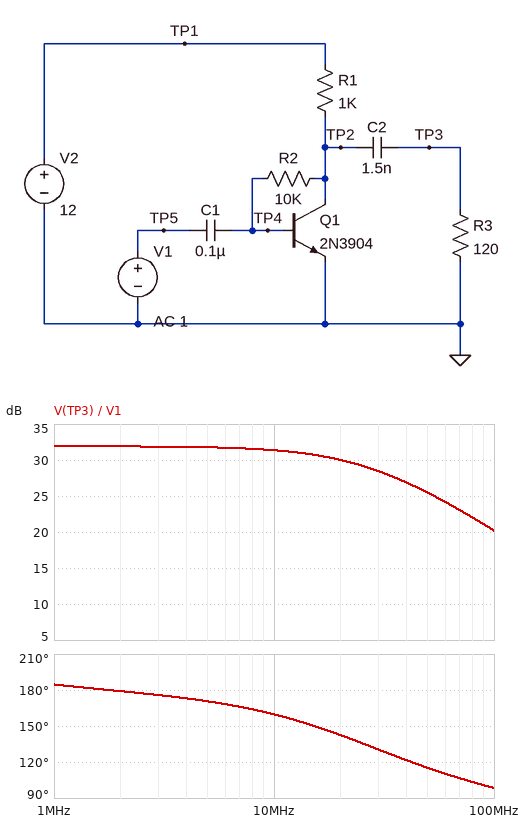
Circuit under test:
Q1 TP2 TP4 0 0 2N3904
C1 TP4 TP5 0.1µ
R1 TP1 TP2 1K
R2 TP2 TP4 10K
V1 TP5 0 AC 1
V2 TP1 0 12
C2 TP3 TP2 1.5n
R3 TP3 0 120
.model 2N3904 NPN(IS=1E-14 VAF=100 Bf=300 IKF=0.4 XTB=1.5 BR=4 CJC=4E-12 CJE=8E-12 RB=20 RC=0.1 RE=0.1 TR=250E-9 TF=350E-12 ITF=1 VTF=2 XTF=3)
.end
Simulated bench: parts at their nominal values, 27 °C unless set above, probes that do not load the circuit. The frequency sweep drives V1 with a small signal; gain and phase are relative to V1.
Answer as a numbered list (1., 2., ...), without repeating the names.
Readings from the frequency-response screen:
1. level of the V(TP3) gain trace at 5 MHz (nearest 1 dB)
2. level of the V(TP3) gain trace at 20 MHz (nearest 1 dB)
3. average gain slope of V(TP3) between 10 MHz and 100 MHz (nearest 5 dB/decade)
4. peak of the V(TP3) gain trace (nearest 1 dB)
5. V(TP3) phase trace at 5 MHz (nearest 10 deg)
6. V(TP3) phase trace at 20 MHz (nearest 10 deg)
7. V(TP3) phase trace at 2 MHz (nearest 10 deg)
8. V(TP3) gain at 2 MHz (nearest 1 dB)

1. 32 dB
2. 30 dB
3. -10 dB/decade
4. 32 dB
5. 170 deg
6. 140 deg
7. 180 deg
8. 32 dB
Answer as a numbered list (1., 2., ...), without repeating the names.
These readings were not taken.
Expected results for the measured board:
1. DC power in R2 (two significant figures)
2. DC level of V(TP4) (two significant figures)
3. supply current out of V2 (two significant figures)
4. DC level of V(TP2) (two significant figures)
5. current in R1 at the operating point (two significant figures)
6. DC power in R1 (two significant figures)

1. 14 µW
2. 720 mV
3. 11 mA
4. 1.1 V
5. 11 mA
6. 120 mW
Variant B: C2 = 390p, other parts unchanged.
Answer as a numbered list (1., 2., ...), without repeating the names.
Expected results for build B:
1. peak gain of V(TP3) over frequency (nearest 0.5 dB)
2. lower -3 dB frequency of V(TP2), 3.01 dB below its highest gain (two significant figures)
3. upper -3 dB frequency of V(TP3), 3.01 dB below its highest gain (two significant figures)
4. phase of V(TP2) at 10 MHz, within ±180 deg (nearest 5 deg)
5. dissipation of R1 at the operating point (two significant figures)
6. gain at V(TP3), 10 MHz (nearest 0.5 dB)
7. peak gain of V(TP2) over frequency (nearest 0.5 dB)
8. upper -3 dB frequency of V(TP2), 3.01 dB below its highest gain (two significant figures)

1. 31.5 dB
2. 46 kHz
3. 29 MHz
4. 145 deg
5. 120 mW
6. 31.0 dB
7. 50.0 dB
8. 470 kHz
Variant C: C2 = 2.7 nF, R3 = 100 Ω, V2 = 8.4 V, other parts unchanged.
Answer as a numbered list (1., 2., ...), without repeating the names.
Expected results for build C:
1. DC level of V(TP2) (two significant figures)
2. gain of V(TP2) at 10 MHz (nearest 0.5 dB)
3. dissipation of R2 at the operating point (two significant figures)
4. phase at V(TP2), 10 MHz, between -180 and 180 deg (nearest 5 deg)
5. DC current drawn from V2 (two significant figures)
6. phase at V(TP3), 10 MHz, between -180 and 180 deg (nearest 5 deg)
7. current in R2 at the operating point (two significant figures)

1. 960 mV
2. 27.5 dB
3. 6.3 µW
4. 160 deg
5. 7.4 mA
6. 165 deg
7. 25 µA
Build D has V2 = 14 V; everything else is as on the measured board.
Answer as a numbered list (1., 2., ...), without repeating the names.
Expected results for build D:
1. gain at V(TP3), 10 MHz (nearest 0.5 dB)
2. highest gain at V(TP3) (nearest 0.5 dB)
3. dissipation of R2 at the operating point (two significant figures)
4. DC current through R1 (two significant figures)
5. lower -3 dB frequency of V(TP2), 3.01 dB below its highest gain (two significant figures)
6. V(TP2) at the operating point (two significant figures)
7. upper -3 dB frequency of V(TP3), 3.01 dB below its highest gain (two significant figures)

1. 32.5 dB
2. 33.0 dB
3. 19 µW
4. 13 mA
5. 41 kHz
6. 1.2 V
7. 24 MHz
